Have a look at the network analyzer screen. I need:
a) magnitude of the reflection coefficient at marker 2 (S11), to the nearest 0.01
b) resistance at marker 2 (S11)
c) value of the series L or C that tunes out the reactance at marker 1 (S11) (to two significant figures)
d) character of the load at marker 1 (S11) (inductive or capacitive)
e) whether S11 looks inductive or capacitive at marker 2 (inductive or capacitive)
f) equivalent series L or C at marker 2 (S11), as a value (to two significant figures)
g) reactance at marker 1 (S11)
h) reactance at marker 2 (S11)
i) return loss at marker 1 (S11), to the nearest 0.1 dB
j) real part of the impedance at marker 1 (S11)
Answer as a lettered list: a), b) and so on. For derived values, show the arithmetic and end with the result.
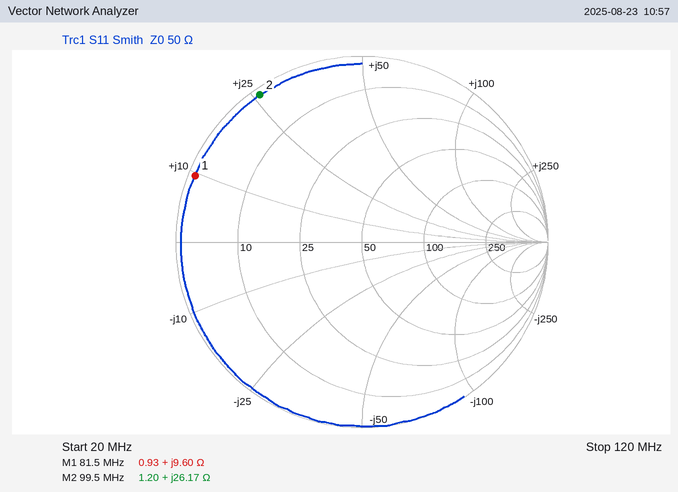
a) 0.96
b) 1.20 Ω
c) C = 1/(2π × 81.5 MHz × 9.6 Ω) ≈ 203 pF, so 200 pF to two significant figures
d) inductive
e) inductive
f) L = 26.17 Ω/(2π × 99.5 MHz) ≈ 42 nH
g) +9.60 Ω
h) +26.17 Ω
i) 0.3 dB
j) 0.93 Ω
